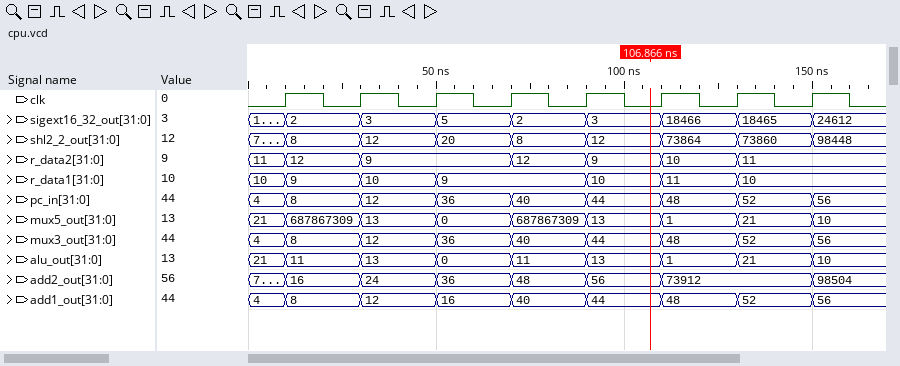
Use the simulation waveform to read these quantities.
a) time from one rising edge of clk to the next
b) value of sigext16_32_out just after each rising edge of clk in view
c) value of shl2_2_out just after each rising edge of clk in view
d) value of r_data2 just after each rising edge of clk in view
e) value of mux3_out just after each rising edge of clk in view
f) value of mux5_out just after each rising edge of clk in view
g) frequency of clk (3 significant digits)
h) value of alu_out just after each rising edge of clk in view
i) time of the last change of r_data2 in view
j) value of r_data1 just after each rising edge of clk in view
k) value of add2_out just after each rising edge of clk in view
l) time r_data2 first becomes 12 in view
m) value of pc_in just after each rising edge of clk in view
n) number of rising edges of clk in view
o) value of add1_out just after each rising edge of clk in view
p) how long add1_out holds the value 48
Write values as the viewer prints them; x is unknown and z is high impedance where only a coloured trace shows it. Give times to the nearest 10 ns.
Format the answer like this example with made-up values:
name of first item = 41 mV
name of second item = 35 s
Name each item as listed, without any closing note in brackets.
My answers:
time from one rising edge of clk to the next = 20 ns
value of sigext16_32_out just after each rising edge of clk in view = 2, 3, 5, 2, 3, 18466, 18465, 24612
value of shl2_2_out just after each rising edge of clk in view = 8, 12, 20, 8, 12, 73864, 73860, 98448
value of r_data2 just after each rising edge of clk in view = 12, 9, 9, 12, 9, 10, 11, 11
value of mux3_out just after each rising edge of clk in view = 8, 12, 36, 40, 44, 48, 52, 56
value of mux5_out just after each rising edge of clk in view = 687867309, 13, 0, 687867309, 13, 1, 21, 10
frequency of clk = 50.0 MHz
value of alu_out just after each rising edge of clk in view = 11, 13, 0, 11, 13, 1, 21, 10
time of the last change of r_data2 in view = 130 ns
value of r_data1 just after each rising edge of clk in view = 9, 10, 9, 9, 10, 11, 10, 10
value of add2_out just after each rising edge of clk in view = 16, 24, 36, 48, 56, 73912, 73912, 98504
time r_data2 first becomes 12 in view = 10 ns
value of pc_in just after each rising edge of clk in view = 8, 12, 36, 40, 44, 48, 52, 56
number of rising edges of clk in view = 8
value of add1_out just after each rising edge of clk in view = 8, 12, 16, 40, 44, 48, 52, 56
how long add1_out holds the value 48 = 20 ns
